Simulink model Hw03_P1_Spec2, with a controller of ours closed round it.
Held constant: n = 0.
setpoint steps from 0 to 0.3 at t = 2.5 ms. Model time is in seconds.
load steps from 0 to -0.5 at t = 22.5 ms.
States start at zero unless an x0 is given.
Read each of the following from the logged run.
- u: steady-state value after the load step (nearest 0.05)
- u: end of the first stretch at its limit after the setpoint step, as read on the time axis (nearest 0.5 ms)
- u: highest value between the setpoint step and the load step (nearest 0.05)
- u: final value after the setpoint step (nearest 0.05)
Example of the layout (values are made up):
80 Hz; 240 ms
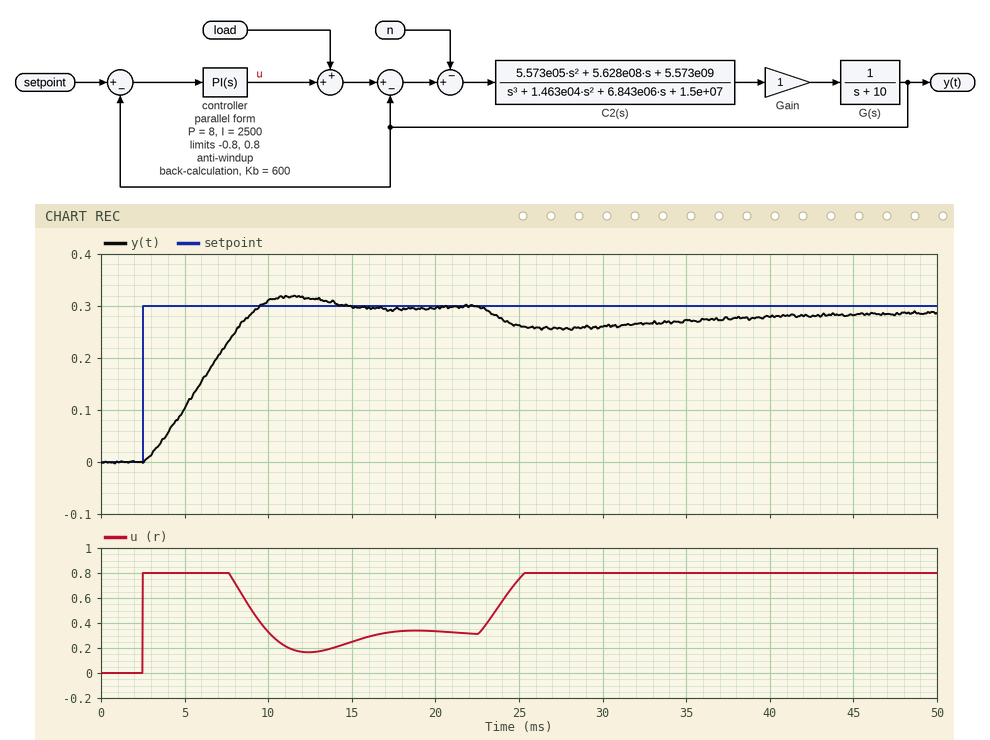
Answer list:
0.80; 7.5 ms; 0.80; 0.30
